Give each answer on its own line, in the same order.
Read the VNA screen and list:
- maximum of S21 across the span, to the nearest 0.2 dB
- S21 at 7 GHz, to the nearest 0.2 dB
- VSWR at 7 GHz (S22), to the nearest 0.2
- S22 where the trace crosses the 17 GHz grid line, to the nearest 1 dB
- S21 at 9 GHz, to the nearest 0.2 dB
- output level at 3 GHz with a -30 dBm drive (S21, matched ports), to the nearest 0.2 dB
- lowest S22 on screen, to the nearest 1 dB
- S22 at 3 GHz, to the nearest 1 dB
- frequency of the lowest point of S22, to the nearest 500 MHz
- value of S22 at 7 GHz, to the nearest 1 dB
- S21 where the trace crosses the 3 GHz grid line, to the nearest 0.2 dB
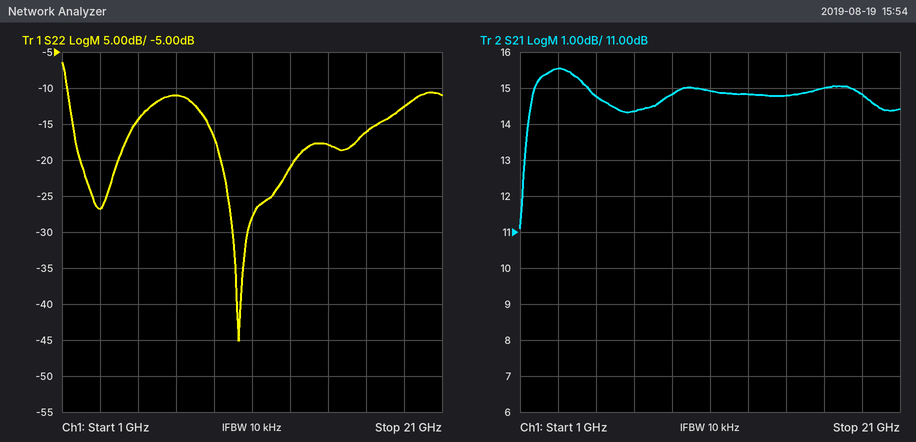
15.6 dB
14.4 dB
1.8
-16 dB
14.8 dB
-14.4 dBm
-45 dB
-27 dB
10.5 GHz
-11 dB
15.6 dB
